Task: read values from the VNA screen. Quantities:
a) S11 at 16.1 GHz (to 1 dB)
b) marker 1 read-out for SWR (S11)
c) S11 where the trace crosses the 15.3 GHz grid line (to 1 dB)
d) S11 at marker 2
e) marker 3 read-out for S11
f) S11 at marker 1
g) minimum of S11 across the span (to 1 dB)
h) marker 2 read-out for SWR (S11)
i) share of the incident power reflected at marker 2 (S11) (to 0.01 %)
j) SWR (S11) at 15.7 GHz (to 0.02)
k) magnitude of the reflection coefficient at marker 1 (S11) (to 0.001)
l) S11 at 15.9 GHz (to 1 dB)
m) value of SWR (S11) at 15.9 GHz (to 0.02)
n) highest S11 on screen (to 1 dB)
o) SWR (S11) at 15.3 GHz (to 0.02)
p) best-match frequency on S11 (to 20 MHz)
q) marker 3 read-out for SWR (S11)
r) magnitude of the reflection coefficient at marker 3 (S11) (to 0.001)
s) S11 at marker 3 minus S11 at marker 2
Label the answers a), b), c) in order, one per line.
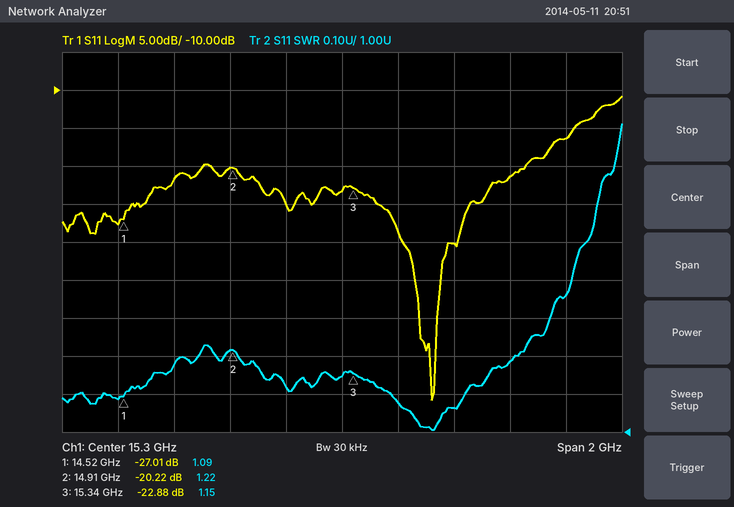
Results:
a) -16 dB
b) 1.09
c) -23 dB
d) -20.22 dB
e) -22.88 dB
f) -27.01 dB
g) -51 dB
h) 1.22
i) 0.95 %
j) 1.06
k) 0.045
l) -21 dB
m) 1.18
n) -11 dB
o) 1.14
p) 15.62 GHz
q) 1.15
r) 0.072
s) -2.66 dB
